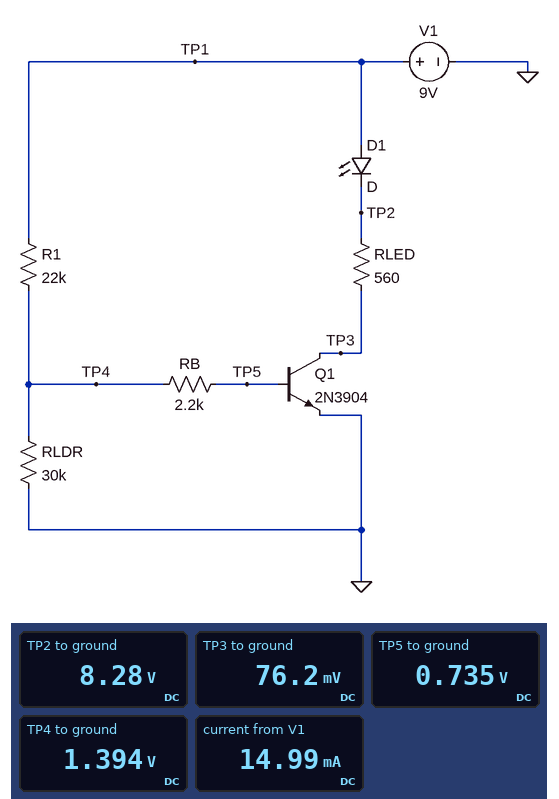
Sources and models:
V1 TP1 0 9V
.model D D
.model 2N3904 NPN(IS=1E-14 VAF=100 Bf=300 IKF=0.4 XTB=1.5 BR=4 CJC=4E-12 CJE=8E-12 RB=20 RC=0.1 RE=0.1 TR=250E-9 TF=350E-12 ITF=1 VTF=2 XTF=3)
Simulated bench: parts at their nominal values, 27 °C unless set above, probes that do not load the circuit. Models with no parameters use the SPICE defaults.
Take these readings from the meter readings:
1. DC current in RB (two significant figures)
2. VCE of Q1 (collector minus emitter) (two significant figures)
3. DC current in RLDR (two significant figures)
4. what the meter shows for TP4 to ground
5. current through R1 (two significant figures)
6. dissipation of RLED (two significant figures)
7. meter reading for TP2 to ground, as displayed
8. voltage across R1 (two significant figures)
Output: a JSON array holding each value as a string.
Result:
["300 µA", "76 mV", "46 µA", "1.394 V", "350 µA", "120 mW", "8.28 V", "7.6 V"]
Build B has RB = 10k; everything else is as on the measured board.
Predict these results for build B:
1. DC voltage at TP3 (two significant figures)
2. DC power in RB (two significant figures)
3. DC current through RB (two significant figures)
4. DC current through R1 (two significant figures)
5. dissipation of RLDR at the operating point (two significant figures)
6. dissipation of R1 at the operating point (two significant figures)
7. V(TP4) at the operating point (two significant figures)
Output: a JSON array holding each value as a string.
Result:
["89 mV", "390 µW", "200 µA", "290 µA", "240 µW", "1.8 mW", "2.7 V"]
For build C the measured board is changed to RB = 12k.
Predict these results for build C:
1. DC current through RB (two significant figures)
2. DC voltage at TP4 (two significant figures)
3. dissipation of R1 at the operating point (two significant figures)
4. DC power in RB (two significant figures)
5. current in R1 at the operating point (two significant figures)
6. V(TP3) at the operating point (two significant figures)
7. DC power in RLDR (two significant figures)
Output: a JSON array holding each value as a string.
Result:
["180 µA", "2.9 V", "1.7 mW", "390 µW", "280 µA", "92 mV", "280 µW"]
